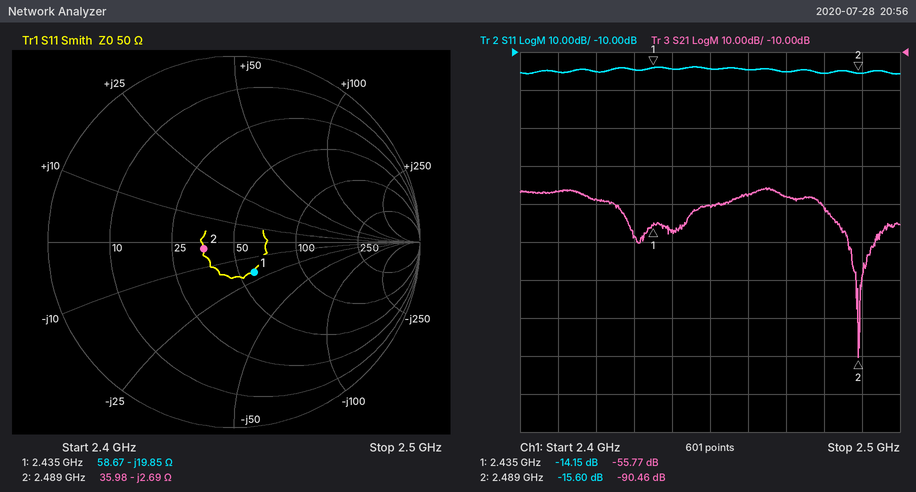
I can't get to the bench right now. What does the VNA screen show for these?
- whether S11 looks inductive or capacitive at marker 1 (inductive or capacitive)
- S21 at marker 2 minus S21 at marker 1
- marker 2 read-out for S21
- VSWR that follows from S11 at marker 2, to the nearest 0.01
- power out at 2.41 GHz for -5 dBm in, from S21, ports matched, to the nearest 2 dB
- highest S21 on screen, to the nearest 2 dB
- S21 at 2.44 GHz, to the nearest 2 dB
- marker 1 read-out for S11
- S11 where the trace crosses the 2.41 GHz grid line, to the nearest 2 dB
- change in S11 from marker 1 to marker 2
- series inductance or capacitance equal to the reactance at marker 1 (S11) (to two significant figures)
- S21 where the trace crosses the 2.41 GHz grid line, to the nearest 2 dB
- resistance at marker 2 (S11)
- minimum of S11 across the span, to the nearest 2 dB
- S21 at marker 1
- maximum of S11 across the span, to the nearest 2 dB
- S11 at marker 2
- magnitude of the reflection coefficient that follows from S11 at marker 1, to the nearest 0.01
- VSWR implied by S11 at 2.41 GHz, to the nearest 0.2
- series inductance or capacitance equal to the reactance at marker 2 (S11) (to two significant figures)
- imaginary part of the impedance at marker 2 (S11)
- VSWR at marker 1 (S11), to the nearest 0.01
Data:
capacitive
-34.69 dB
-90.46 dB
1.40
-52 dBm
-46 dB
-56 dB
-14.15 dB
-16 dB
-1.45 dB
3.3 pF
-46 dB
35.98 Ω
-16 dB
-55.77 dB
-14 dB
-15.60 dB
0.20
1.4
24 pF
-2.69 Ω
1.49
